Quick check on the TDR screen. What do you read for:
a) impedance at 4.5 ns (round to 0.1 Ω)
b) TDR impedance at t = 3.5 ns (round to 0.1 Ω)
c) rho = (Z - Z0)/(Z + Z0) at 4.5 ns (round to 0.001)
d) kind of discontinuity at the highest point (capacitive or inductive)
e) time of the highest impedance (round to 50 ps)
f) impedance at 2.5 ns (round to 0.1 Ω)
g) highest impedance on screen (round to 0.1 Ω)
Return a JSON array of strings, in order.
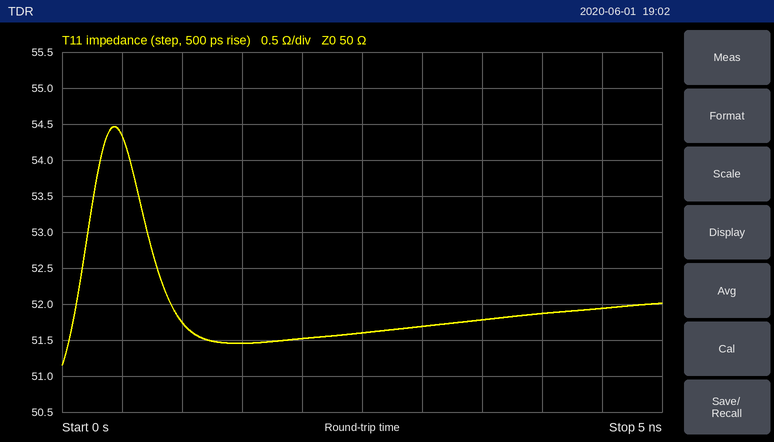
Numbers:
["51.9 Ω", "51.8 Ω", "+0.019", "inductive", "450 ps", "51.6 Ω", "54.5 Ω"]
